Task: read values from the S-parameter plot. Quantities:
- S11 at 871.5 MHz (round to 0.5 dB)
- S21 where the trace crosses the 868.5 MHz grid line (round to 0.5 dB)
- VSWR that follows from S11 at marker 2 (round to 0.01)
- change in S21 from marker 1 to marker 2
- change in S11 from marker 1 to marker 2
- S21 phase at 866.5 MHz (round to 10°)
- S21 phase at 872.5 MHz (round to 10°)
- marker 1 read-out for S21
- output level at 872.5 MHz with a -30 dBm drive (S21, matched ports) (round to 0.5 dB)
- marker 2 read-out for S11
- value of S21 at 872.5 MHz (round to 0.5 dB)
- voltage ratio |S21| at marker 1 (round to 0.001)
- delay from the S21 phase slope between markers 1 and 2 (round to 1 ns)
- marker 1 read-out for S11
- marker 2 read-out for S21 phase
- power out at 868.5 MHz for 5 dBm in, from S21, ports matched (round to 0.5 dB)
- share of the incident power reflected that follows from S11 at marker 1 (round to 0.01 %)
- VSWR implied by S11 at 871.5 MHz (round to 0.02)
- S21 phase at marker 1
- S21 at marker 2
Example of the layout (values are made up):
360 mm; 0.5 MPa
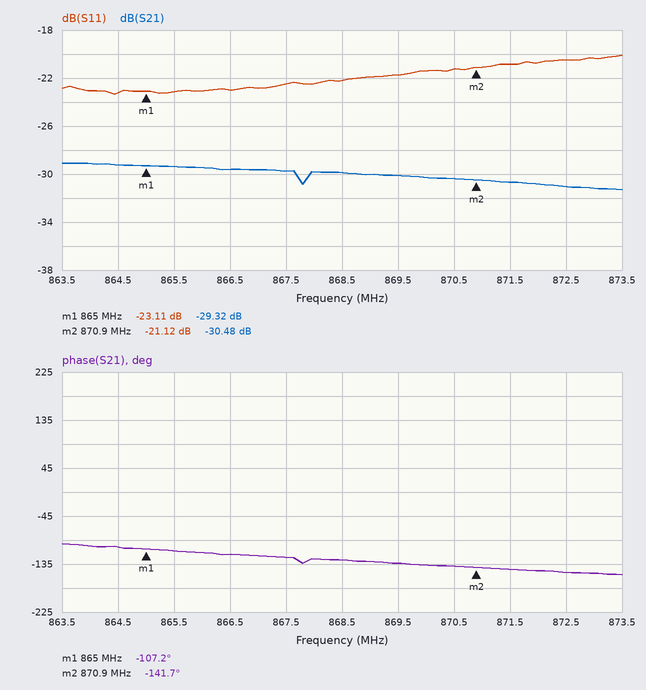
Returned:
-21.0 dB; -30.0 dB; 1.19; -1.16 dB; 1.99 dB; -120°; -150°; -29.32 dB; -61.0 dBm; -21.12 dB; -31.0 dB; 0.034; 16 ns; -23.11 dB; -141.7°; -25.0 dBm; 0.49 %; 1.20; -107.2°; -30.48 dB
